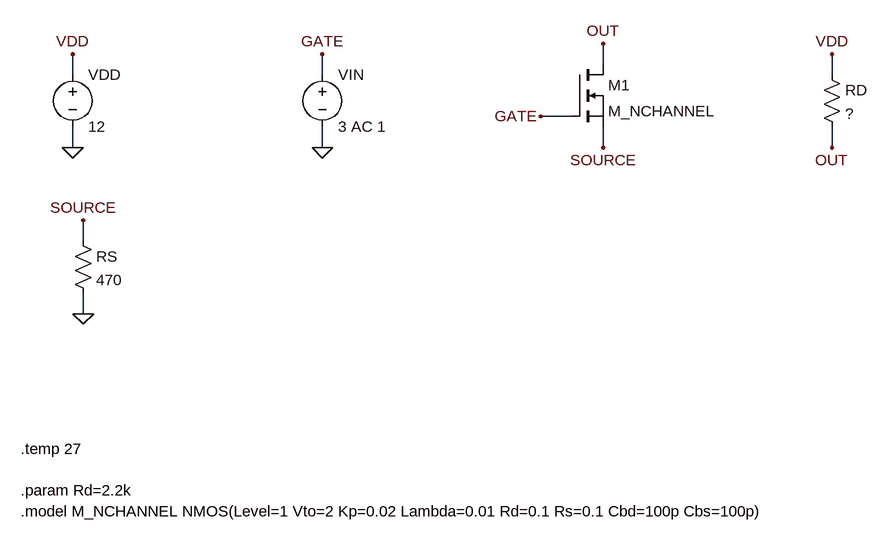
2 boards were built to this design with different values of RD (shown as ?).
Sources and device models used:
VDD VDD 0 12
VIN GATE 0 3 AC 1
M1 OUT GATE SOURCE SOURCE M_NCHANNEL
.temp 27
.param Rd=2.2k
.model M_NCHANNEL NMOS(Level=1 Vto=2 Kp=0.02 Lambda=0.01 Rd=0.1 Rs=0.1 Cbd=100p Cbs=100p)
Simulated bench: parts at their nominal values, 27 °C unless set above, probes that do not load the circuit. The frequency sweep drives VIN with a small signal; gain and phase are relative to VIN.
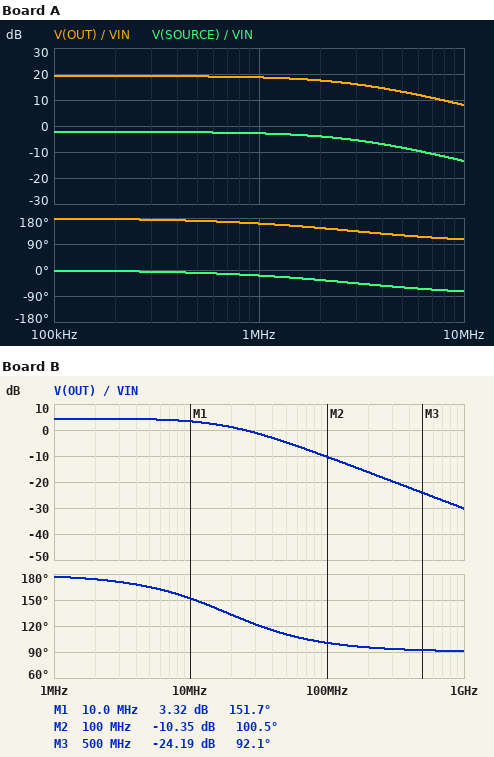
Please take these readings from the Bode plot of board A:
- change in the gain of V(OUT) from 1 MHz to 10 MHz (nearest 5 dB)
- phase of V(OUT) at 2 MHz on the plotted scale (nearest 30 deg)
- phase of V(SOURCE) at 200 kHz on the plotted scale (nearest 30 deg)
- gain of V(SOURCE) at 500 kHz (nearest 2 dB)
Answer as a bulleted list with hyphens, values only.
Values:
- -10 dB
- 150 deg
- 0 deg
- -2 dB
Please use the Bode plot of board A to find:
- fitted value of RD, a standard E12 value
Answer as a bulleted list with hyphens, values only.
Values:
- 5.6 kΩ
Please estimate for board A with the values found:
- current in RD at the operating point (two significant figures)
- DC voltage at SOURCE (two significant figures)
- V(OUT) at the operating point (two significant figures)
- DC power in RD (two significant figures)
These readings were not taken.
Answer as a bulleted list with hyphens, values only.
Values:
- 1.4 mA
- 640 mV
- 4.4 V
- 10 mW
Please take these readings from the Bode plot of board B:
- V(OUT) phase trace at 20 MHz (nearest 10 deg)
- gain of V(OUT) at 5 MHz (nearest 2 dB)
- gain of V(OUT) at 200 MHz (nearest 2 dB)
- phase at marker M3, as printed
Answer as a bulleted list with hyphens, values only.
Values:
- 130 deg
- 4 dB
- -16 dB
- 92.1 deg
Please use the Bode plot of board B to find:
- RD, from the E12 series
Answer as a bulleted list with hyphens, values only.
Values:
- 1 kΩ
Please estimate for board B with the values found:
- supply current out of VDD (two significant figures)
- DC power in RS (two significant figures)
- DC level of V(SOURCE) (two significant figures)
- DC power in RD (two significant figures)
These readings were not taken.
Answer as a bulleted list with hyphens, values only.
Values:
- 1.4 mA
- 890 µW
- 650 mV
- 1.9 mW
